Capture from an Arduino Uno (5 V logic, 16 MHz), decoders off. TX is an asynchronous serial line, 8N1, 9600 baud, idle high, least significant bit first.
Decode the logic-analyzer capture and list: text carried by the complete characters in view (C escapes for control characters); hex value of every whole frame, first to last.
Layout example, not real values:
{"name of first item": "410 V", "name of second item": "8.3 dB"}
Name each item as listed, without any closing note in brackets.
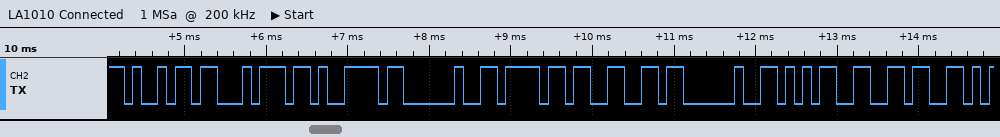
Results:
{"text carried by the complete characters in view": "\"ity of 56\"", "hex value of every whole frame, first to last": "0x69 0x74 0x79 0x20 0x6F 0x66 0x20 0x35 0x36"}
